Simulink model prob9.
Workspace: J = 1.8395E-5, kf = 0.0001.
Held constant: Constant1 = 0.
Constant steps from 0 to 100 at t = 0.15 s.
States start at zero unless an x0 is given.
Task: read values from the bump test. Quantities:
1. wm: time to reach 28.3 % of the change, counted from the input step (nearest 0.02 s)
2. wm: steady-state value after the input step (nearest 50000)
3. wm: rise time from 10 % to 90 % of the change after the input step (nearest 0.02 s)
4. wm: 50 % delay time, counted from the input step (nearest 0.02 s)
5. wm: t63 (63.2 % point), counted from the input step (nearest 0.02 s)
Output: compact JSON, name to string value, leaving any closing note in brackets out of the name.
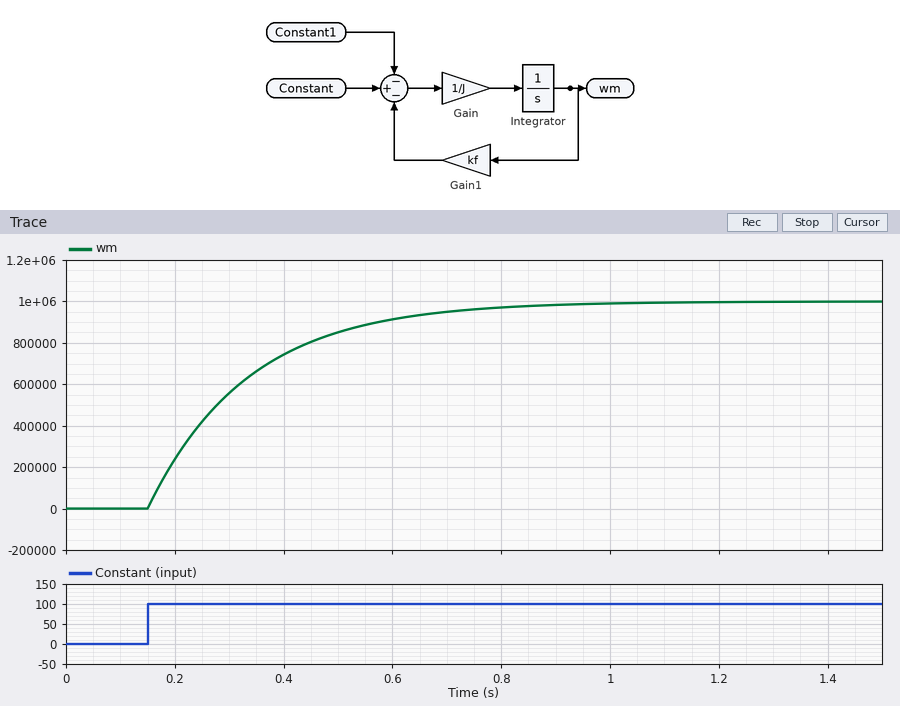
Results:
{"wm: time to reach 28.3 % of the change, counted from the input step": "0.06 s", "wm: steady-state value after the input step": "1000000", "wm: rise time from 10 % to 90 % of the change after the input step": "0.40 s", "wm: 50 % delay time, counted from the input step": "0.12 s", "wm: t63 (63.2 % point), counted from the input step": "0.18 s"}
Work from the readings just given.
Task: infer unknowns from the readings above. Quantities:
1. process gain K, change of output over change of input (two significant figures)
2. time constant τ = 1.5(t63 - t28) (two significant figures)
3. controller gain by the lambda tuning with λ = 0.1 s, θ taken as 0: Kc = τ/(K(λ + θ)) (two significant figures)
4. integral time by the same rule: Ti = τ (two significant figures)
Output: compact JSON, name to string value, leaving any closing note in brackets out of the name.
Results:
{"process gain K, change of output over change of input": "10000", "time constant τ = 1.5(t63 - t28)": "0.18 s", "controller gain by the lambda tuning with λ = 0.1 s, θ taken as 0: Kc = τ/(K(λ + θ))": "0.00018", "integral time by the same rule: Ti = τ": "0.18 s"}
